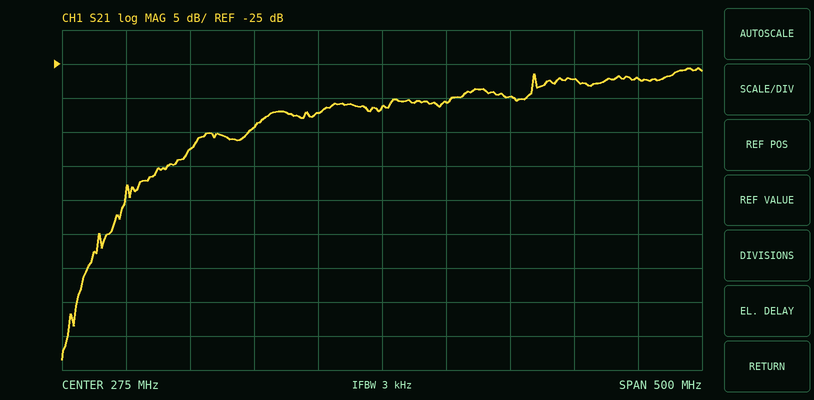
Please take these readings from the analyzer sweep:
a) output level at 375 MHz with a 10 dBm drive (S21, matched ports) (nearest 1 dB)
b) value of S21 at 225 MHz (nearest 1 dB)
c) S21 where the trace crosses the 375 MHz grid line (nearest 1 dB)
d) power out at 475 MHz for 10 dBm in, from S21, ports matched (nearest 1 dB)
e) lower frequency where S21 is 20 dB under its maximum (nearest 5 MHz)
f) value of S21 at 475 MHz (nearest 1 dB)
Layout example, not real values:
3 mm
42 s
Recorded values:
-20 dBm
-32 dB
-30 dB
-17 dBm
75 MHz
-27 dB
